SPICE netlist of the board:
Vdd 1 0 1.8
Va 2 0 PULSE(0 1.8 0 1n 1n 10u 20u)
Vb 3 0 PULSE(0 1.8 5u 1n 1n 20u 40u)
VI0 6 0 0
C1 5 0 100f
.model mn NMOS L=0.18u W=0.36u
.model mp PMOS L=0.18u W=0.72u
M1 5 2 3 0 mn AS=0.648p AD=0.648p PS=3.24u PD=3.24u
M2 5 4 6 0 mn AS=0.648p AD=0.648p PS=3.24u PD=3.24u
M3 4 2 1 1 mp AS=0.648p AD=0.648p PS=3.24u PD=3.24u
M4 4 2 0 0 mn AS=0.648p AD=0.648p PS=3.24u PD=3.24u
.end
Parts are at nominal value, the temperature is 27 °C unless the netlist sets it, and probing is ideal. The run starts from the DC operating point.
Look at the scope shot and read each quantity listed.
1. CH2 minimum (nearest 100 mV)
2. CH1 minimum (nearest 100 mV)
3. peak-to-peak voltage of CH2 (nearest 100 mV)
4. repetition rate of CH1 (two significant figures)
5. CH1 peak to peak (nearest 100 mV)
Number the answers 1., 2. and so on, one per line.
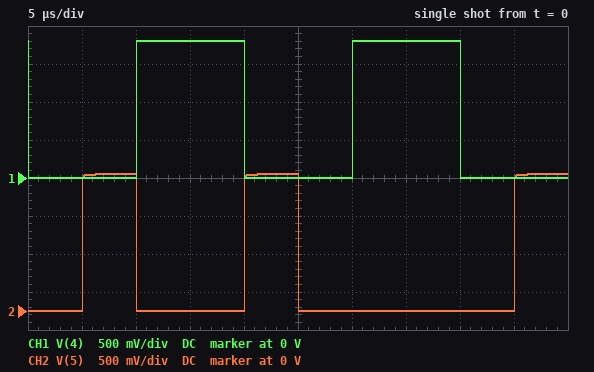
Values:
1. 0 V
2. 0 V
3. 1.8 V
4. 50 kHz
5. 1.8 V
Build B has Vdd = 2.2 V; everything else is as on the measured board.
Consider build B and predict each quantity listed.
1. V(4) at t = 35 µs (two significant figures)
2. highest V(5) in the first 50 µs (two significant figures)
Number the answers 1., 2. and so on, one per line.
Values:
1. 2.2 V
2. 1.7 V
